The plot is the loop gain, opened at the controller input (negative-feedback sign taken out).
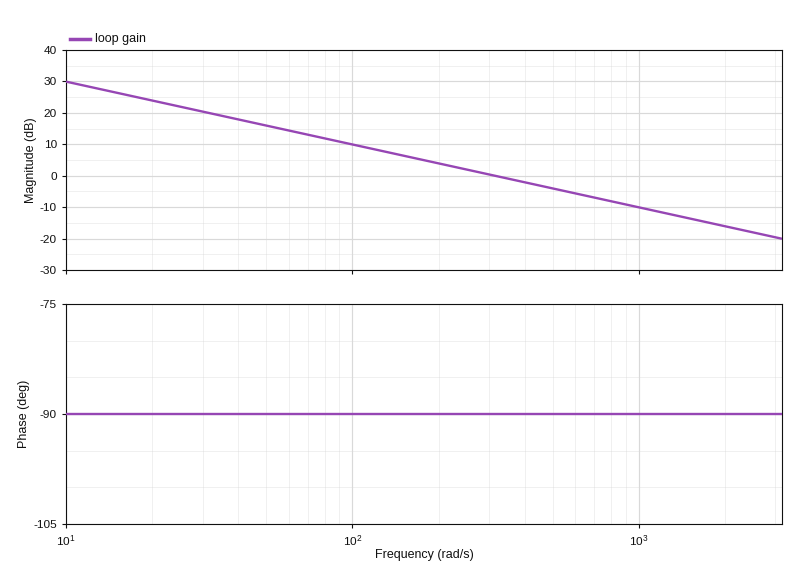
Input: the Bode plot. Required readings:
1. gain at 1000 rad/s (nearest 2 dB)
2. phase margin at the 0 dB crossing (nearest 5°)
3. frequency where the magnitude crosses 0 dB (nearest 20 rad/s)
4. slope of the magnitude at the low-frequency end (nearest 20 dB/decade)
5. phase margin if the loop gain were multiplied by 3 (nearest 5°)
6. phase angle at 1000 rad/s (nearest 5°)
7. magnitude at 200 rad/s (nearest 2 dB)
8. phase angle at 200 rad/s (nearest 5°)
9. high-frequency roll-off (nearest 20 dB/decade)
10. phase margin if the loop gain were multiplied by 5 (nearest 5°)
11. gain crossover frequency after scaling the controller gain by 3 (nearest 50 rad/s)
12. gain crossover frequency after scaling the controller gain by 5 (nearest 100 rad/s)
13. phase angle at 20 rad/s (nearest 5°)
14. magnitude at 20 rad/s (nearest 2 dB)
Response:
-10 dB
90°
320 rad/s
-20 dB/decade
90°
-90°
4 dB
-90°
-20 dB/decade
90°
950 rad/s
1600 rad/s
-90°
24 dB
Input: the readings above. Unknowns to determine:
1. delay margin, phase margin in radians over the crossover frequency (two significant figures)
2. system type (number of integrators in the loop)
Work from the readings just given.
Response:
0.0049 s
1
